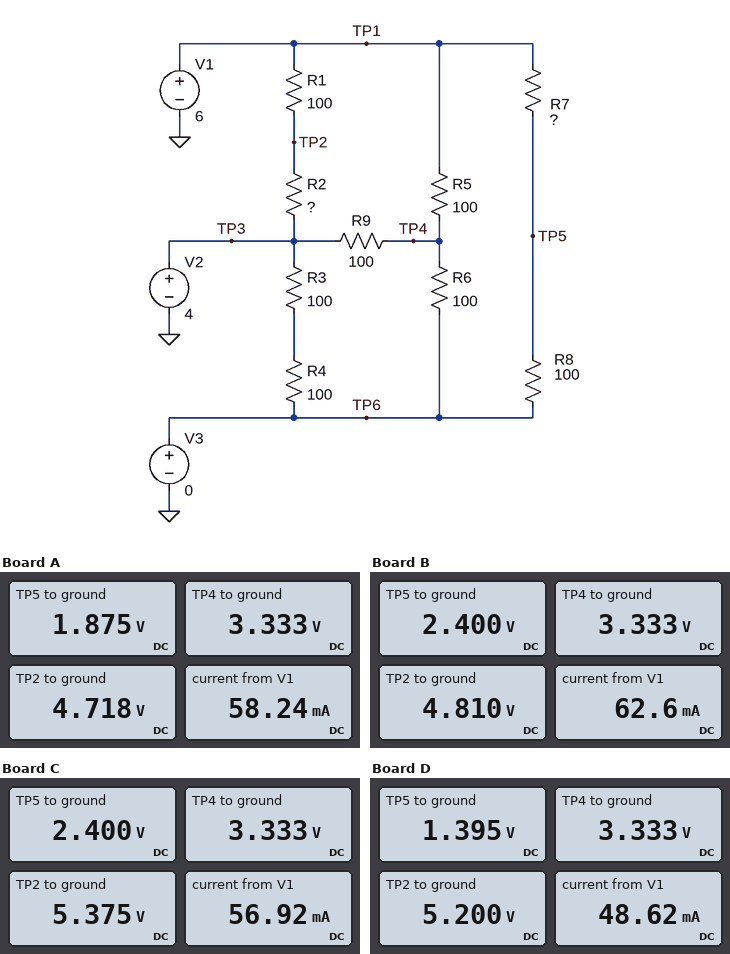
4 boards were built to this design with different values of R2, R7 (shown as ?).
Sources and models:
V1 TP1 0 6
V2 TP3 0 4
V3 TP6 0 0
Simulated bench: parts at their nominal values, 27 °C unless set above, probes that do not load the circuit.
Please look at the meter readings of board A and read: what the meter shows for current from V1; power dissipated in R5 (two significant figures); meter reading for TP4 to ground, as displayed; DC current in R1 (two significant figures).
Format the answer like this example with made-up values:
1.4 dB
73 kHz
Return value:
58.24 mA
71 mW
3.333 V
13 mA
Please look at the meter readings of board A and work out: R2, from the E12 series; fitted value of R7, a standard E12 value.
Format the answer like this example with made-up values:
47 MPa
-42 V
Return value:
56 Ω
220 Ω
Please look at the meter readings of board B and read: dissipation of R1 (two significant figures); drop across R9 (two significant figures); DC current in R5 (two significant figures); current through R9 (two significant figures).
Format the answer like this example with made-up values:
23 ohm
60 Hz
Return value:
14 mW
670 mV
27 mA
6.7 mA
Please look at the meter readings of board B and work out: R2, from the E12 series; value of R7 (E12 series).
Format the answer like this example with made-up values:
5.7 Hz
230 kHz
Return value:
68 Ω
150 Ω
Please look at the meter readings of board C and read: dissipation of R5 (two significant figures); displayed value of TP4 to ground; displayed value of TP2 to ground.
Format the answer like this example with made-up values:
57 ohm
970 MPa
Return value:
71 mW
3.333 V
5.375 V
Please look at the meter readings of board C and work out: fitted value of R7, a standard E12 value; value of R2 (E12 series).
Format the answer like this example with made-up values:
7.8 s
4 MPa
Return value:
150 Ω
220 Ω
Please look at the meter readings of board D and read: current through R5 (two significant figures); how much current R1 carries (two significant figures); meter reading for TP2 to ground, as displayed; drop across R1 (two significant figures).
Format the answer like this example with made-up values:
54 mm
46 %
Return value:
27 mA
8.0 mA
5.200 V
800 mV
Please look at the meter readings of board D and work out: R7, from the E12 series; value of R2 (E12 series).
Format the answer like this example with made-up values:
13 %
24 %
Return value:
330 Ω
150 Ω
